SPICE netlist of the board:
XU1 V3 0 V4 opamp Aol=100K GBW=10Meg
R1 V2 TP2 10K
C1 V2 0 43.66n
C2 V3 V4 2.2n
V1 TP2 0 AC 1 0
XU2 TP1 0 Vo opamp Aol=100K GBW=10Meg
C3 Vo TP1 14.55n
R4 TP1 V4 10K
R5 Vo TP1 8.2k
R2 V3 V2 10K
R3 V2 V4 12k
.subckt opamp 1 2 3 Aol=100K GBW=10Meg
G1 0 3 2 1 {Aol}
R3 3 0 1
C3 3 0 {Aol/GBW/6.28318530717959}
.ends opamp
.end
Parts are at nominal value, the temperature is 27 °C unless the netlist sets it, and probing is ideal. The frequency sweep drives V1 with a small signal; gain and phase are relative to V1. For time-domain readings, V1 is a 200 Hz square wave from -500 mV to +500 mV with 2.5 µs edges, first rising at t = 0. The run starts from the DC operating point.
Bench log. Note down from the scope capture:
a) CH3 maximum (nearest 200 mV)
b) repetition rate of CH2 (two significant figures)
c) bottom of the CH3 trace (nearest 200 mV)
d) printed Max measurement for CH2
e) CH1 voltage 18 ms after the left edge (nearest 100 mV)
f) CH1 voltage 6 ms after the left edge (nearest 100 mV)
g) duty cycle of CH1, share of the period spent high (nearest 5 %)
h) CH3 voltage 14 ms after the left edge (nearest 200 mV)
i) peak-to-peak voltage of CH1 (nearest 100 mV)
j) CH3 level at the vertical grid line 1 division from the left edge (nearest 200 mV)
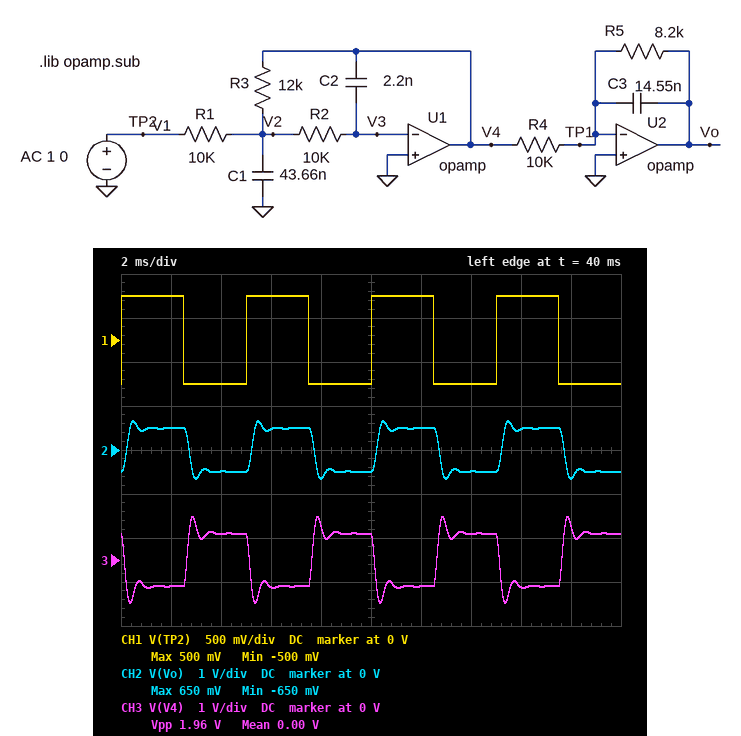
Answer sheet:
1.0 V
200 Hz
-1.0 V
650 mV
-500 mV
500 mV
50 %
600 mV
1.0 V
-600 mV
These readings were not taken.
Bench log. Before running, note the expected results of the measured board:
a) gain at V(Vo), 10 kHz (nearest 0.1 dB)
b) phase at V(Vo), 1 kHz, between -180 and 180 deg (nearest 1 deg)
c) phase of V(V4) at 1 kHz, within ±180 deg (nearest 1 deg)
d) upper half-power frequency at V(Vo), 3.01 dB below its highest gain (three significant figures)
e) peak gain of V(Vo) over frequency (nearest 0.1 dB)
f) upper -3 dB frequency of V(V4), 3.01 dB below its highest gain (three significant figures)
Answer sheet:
-50.7 dB
-78 deg
139 deg
1.63 kHz
0.9 dB
1.76 kHz
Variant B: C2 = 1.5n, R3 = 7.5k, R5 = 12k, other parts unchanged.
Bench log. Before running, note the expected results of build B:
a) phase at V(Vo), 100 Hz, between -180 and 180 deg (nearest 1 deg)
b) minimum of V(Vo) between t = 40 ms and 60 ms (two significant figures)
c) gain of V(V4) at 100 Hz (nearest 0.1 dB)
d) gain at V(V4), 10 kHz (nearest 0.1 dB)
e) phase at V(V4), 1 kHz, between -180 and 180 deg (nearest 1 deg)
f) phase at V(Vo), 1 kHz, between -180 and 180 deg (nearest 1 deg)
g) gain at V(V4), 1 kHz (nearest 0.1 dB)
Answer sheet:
-8 deg
-460 mV
-2.5 dB
-27.9 dB
164 deg
-64 deg
-1.0 dB
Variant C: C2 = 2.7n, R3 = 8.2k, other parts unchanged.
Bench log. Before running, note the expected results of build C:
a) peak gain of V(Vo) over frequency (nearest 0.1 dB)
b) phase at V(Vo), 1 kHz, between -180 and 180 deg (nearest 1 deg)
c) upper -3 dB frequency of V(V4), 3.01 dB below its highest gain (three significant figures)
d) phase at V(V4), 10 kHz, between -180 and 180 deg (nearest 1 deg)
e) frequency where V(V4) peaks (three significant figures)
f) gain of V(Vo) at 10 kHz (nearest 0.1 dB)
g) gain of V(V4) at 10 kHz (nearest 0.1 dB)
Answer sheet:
-2.9 dB
-73 deg
1.92 kHz
7 deg
1.39 kHz
-52.5 dB
-33.2 dB
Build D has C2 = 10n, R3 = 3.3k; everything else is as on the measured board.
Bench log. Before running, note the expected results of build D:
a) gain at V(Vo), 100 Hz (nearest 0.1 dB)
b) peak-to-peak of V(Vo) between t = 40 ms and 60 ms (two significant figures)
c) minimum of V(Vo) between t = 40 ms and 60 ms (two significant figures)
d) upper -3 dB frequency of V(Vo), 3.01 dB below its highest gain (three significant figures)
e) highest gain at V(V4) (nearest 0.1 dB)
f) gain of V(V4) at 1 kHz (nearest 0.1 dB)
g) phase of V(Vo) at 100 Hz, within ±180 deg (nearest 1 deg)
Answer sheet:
-11.4 dB
280 mV
-140 mV
1.00 kHz
-9.6 dB
-10.7 dB
-10 deg
